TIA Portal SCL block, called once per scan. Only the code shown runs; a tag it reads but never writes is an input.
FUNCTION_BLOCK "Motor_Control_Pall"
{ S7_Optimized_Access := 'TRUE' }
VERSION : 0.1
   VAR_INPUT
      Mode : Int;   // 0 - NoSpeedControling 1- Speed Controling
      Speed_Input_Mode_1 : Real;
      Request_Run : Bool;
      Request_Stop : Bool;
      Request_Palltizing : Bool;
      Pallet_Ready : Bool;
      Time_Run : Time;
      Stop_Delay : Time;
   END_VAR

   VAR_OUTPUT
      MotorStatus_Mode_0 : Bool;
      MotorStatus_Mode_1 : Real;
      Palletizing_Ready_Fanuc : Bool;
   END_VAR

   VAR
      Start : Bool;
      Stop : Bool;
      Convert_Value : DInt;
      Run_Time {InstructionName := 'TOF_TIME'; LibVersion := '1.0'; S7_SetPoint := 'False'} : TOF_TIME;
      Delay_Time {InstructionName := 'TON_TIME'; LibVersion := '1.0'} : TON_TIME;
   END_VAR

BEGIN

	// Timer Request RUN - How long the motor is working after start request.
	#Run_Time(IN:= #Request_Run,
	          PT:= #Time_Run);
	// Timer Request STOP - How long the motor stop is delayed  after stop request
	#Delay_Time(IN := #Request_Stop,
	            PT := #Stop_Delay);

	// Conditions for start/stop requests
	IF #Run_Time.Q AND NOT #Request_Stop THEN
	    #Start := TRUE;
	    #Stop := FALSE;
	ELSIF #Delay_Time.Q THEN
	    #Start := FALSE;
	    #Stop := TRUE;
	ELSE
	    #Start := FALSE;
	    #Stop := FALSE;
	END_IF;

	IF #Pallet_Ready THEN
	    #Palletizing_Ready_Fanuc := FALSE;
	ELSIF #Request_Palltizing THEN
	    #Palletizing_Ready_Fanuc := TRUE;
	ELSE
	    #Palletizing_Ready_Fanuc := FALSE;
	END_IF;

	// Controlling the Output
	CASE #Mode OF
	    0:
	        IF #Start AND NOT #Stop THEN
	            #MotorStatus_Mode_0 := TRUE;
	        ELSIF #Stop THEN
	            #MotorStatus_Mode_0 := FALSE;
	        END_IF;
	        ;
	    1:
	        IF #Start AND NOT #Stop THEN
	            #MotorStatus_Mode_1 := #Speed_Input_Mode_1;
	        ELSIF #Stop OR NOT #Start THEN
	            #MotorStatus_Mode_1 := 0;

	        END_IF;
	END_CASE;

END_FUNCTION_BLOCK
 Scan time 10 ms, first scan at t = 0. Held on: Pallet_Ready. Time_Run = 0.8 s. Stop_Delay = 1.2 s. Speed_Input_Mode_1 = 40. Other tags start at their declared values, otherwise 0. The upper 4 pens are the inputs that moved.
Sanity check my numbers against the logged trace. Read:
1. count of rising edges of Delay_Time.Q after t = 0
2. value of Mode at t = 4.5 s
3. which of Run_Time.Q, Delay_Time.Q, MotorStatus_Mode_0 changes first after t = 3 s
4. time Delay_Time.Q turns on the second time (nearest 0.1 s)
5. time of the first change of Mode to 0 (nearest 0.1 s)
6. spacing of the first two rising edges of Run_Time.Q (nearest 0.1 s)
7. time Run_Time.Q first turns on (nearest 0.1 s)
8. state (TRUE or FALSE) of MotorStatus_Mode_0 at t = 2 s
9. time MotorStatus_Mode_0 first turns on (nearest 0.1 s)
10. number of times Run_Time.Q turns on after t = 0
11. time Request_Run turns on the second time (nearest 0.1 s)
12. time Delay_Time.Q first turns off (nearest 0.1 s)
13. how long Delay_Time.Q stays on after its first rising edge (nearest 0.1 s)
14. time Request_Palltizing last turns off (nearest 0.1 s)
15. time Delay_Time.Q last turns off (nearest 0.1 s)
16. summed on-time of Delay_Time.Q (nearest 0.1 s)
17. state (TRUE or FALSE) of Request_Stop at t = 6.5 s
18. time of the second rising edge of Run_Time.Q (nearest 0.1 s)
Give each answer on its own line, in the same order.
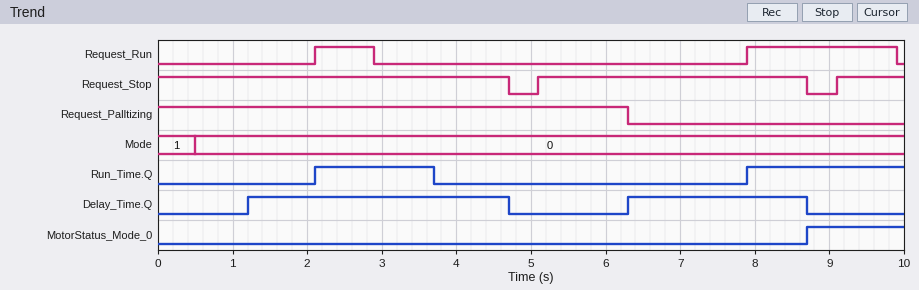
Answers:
2
0
Run_Time.Q
6.3 s
0.5 s
5.8 s
2.1 s
FALSE
8.7 s
2
7.9 s
4.7 s
3.5 s
6.3 s
8.7 s
5.9 s
TRUE
7.9 s
